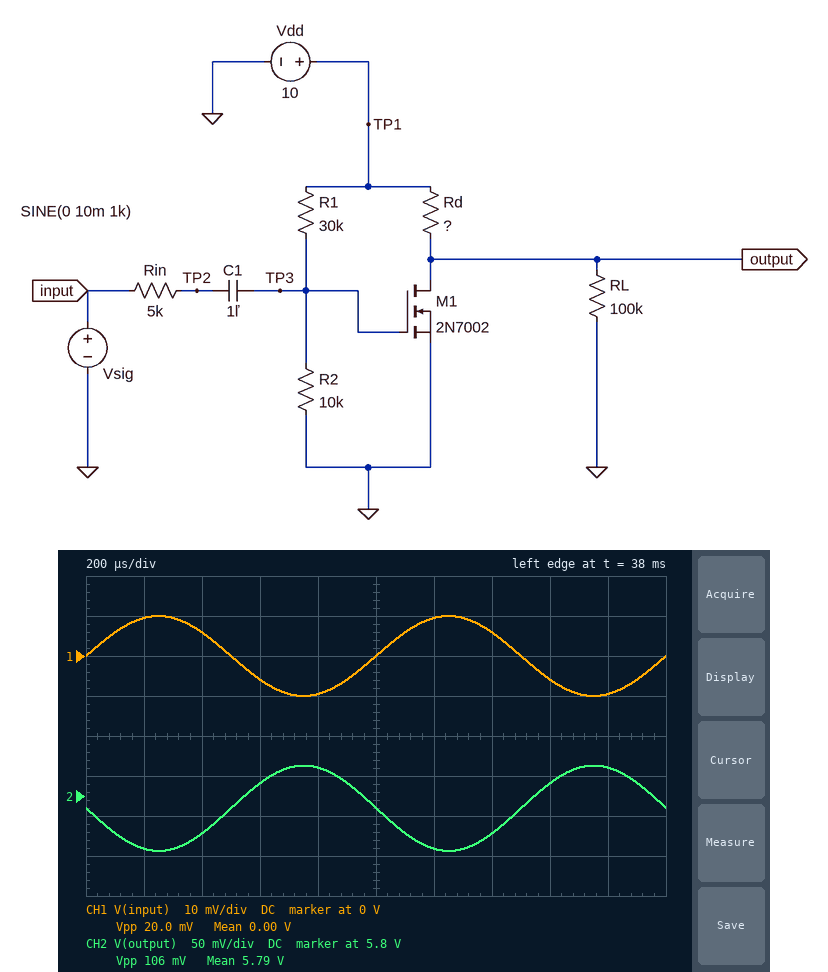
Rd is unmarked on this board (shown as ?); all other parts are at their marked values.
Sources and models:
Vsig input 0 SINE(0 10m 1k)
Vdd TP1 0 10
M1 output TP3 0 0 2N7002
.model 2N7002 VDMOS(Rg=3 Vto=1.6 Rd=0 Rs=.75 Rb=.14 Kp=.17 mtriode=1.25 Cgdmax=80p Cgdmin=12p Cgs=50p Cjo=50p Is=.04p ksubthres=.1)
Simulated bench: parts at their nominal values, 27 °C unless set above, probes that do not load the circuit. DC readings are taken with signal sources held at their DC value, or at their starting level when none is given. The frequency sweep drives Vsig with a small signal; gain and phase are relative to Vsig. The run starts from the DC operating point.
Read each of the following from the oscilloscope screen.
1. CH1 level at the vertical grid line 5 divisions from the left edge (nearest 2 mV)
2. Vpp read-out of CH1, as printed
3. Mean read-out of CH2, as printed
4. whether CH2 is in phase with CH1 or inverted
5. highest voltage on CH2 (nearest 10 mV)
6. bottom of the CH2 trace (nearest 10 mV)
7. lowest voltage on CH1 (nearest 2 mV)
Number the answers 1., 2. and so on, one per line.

1. 0 V
2. 20.0 mV
3. 5.79 V
4. inverted
5. 5.84 V
6. 5.73 V
7. -10 mV
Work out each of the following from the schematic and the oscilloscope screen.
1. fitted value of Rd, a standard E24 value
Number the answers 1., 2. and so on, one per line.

1. 68 Ω
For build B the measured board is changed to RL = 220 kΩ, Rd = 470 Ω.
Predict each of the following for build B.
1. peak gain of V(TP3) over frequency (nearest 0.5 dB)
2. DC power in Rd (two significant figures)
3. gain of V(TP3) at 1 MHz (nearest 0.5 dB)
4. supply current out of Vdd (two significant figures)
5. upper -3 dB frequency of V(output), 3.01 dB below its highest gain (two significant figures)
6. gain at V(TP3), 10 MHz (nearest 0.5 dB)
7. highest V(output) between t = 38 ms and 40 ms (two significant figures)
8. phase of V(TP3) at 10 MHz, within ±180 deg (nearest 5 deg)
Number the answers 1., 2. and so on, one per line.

1. -4.5 dB
2. 210 mW
3. -13.5 dB
4. 21 mA
5. 370 kHz
6. -33.0 dB
7. 140 mV
8. -85 deg
